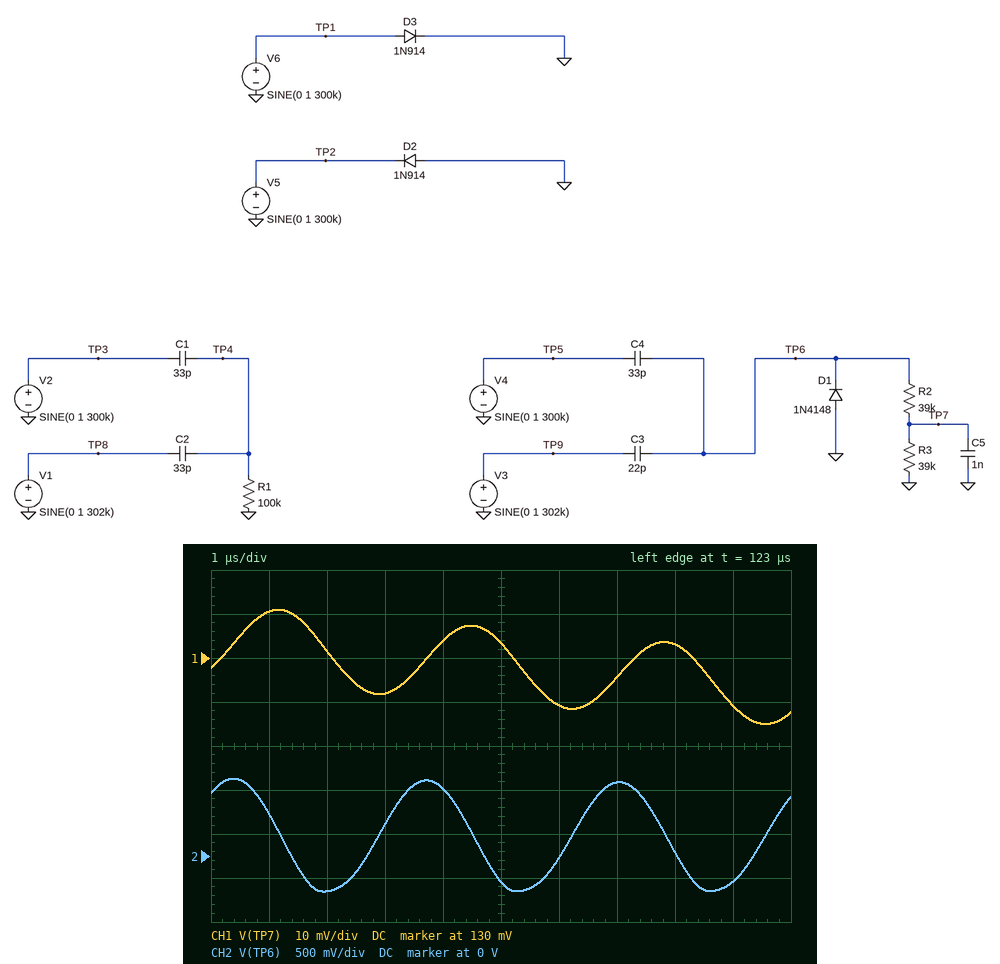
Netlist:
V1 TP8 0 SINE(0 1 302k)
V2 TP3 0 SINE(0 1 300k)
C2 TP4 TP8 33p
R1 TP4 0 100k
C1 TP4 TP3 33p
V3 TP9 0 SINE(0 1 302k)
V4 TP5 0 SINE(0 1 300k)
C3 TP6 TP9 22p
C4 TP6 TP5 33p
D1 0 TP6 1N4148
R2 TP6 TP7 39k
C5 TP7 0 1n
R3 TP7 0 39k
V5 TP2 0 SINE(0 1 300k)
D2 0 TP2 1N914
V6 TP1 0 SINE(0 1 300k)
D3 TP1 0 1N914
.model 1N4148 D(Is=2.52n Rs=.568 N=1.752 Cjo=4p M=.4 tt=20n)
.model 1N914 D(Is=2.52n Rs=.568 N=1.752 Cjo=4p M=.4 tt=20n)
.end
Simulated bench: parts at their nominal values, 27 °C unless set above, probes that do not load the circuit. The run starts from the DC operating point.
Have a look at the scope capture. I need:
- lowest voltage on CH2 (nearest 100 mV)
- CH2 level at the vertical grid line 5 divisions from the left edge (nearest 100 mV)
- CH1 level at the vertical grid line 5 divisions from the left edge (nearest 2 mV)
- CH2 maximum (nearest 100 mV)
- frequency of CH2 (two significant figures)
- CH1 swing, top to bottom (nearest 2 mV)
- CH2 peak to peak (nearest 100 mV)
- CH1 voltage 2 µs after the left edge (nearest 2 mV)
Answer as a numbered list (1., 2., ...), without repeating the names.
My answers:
1. -400 mV
2. -300 mV
3. 134 mV
4. 900 mV
5. 300 kHz
6. 26 mV
7. 1.3 V
8. 132 mV
